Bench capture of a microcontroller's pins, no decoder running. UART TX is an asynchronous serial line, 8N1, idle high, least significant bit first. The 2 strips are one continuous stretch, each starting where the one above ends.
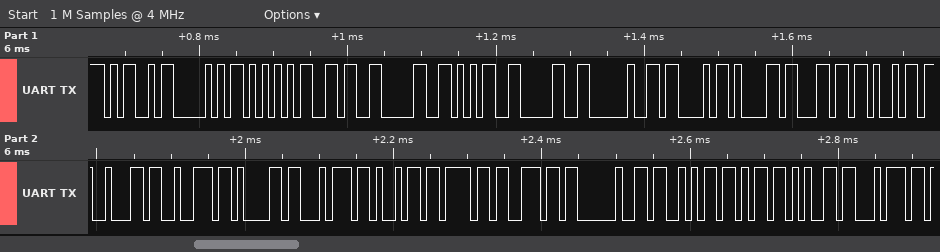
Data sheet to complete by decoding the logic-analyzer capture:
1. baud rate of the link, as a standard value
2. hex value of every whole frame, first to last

115200 baud
0x4D 0x50 0x55 0x36 0x30 0x35 0x30 0x20 0x43 0x61 0x6C 0x69 0x62 0x72 0x61 0x74 0x69 0x6F 0x6E 0x20 0x53 0x6B 0x65 0x74
